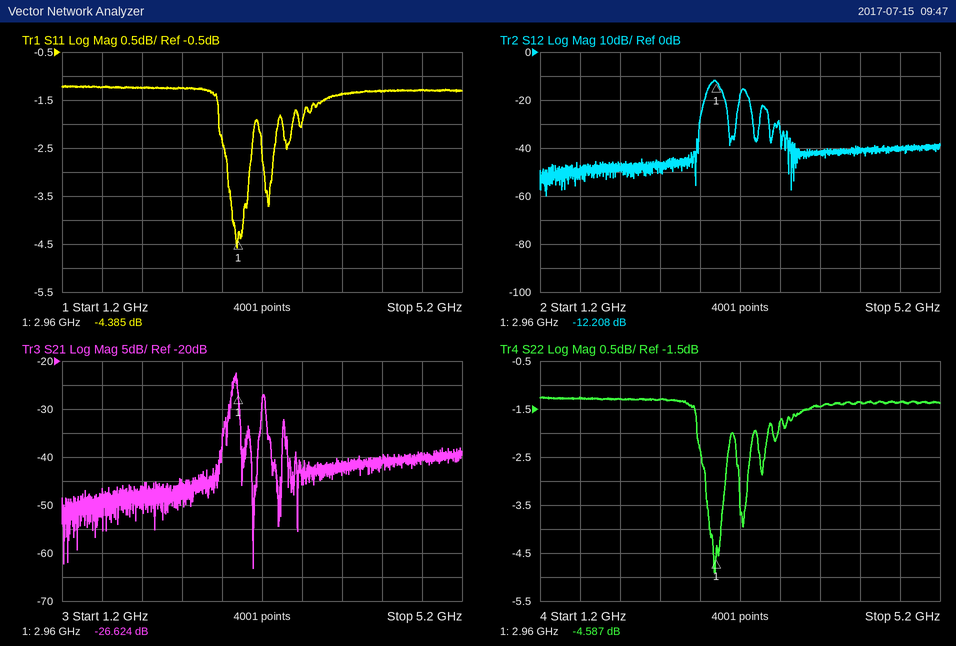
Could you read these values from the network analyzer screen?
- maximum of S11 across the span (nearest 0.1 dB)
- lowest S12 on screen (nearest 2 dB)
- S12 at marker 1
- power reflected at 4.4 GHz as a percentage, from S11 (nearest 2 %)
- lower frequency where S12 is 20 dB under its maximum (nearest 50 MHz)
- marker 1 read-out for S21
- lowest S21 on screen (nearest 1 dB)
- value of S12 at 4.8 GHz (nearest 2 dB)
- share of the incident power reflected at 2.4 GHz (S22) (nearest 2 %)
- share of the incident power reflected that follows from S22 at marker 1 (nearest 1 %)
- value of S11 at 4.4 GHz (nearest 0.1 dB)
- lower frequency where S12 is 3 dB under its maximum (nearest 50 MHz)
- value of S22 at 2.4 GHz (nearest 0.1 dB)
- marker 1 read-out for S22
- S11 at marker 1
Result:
-1.2 dB
-60 dB
-12.208 dB
74 %
2.80 GHz
-26.624 dB
-63 dB
-40 dB
74 %
35 %
-1.3 dB
2.90 GHz
-1.3 dB
-4.587 dB
-4.385 dB
